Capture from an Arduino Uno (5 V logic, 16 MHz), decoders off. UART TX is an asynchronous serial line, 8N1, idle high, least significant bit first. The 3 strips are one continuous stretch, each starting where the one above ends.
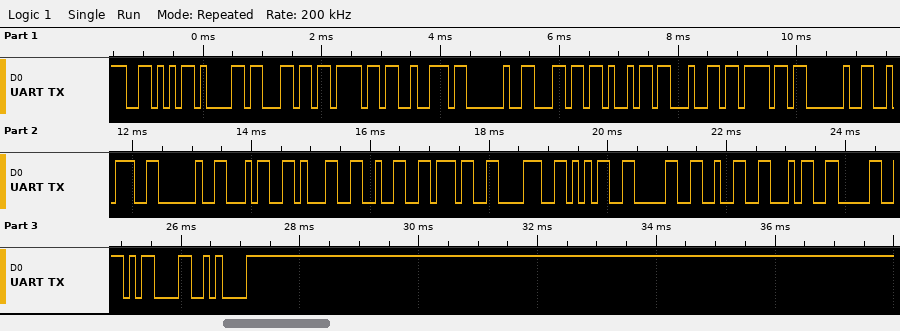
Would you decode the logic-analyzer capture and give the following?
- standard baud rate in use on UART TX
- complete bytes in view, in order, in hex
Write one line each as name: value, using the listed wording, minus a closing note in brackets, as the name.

standard baud rate in use on UART TX: 9600 baud
complete bytes in view, in order, in hex: 56 61 6C 6F 72 20 6C 69 64 6F 20 3A 20 34 31 32 37 38 35 30 32 34 30 0D 0A
